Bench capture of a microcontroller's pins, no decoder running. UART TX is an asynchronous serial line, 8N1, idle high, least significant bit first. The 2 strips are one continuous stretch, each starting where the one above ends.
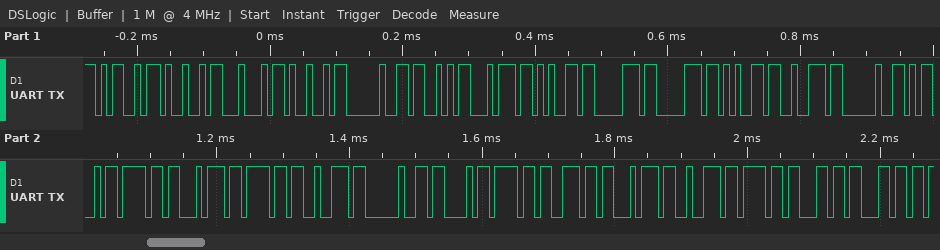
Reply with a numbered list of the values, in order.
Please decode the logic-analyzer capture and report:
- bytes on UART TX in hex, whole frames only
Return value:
1. 0x4D 0x49 0x44 0x49 0x20 0x53 0x74 0x65 0x70 0x70 0x65 0x72 0x20 0x4D 0x6F 0x74 0x6F 0x72 0x20 0x43 0x6F 0x6E 0x74 0x72 0x6F 0x6C 0x6C
